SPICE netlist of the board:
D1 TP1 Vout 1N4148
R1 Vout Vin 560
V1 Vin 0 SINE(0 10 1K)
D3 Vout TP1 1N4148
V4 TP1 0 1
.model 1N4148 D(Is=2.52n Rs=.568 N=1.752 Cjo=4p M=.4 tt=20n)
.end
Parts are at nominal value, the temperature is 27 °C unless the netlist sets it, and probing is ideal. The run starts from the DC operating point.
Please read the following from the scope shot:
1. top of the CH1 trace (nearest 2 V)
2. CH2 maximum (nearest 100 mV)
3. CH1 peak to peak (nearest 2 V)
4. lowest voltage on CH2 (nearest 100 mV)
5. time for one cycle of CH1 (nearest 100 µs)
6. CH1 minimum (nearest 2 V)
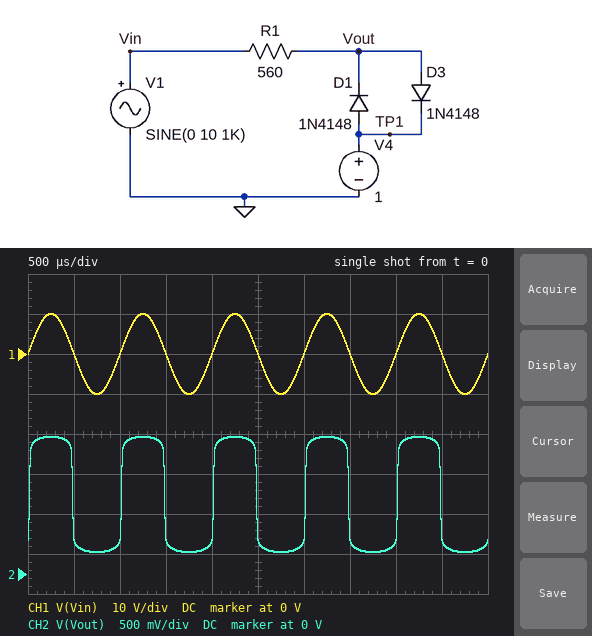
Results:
10 V
1.7 V
20 V
300 mV
1.0 ms
-10 V
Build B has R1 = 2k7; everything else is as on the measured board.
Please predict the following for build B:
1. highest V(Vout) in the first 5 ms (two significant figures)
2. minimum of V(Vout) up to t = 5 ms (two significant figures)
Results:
1.6 V
350 mV
